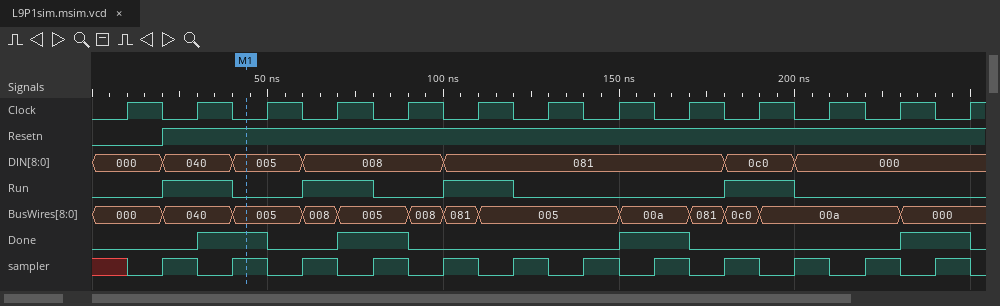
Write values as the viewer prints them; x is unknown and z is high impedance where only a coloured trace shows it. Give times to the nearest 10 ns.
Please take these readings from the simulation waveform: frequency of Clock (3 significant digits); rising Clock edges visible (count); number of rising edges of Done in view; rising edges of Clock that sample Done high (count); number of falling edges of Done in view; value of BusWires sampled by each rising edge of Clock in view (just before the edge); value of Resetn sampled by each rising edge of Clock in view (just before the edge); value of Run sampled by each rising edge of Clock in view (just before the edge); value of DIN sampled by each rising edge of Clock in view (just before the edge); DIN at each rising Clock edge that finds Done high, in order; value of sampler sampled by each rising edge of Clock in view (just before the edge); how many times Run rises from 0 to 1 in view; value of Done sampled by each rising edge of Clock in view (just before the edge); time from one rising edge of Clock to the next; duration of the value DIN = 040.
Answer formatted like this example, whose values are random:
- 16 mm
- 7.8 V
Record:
- 50.0 MHz
- 13
- 4
- 4
- 4
- 000, 040, 005, 008, 005, 081, 005, 005, 00a, 0c0, 00a, 00a, 000
- 0 1 1 1 1 1 1 1 1 1 1 1 1
- 0 1 0 1 0 1 0 0 0 1 0 0 0
- 000, 040, 005, 008, 008, 081, 081, 081, 081, 0c0, 000, 000, 000
- 005, 008, 081, 000
- x 1 1 1 1 1 1 1 1 1 1 1 1
- 4
- 0 0 1 0 1 0 0 0 1 0 0 0 1
- 20 ns
- 20 ns
